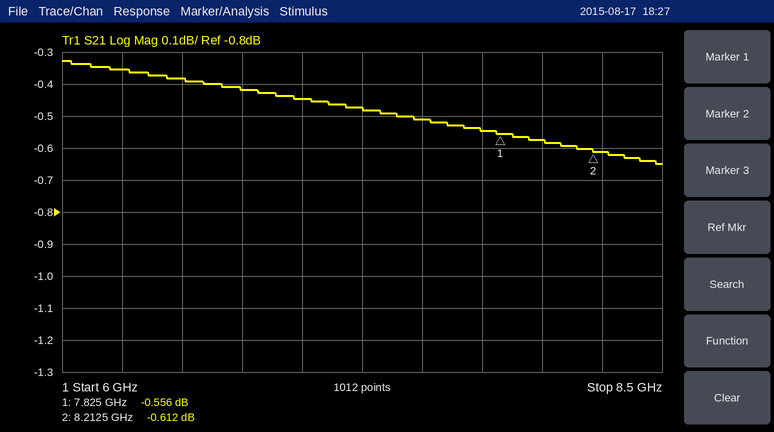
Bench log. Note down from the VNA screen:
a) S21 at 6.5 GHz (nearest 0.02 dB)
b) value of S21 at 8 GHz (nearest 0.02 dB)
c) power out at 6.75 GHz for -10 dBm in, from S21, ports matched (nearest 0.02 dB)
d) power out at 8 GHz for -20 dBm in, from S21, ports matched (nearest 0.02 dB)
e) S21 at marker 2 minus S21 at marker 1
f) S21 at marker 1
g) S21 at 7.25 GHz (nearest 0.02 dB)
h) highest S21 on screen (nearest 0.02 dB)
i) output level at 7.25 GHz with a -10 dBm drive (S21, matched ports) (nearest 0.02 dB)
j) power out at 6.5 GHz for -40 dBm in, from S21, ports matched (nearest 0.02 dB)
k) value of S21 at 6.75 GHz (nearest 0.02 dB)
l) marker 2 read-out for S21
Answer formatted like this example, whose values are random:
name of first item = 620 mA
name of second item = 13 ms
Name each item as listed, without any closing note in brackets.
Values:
S21 at 6.5 GHz = -0.38 dB
value of S21 at 8 GHz = -0.58 dB
power out at 6.75 GHz for -10 dBm in, from S21, ports matched = -10.42 dBm
power out at 8 GHz for -20 dBm in, from S21, ports matched = -20.58 dBm
S21 at marker 2 minus S21 at marker 1 = -0.056 dB
S21 at marker 1 = -0.556 dB
S21 at 7.25 GHz = -0.48 dB
highest S21 on screen = -0.32 dB
output level at 7.25 GHz with a -10 dBm drive (S21, matched ports) = -10.48 dBm
power out at 6.5 GHz for -40 dBm in, from S21, ports matched = -40.38 dBm
value of S21 at 6.75 GHz = -0.42 dB
marker 2 read-out for S21 = -0.612 dB
